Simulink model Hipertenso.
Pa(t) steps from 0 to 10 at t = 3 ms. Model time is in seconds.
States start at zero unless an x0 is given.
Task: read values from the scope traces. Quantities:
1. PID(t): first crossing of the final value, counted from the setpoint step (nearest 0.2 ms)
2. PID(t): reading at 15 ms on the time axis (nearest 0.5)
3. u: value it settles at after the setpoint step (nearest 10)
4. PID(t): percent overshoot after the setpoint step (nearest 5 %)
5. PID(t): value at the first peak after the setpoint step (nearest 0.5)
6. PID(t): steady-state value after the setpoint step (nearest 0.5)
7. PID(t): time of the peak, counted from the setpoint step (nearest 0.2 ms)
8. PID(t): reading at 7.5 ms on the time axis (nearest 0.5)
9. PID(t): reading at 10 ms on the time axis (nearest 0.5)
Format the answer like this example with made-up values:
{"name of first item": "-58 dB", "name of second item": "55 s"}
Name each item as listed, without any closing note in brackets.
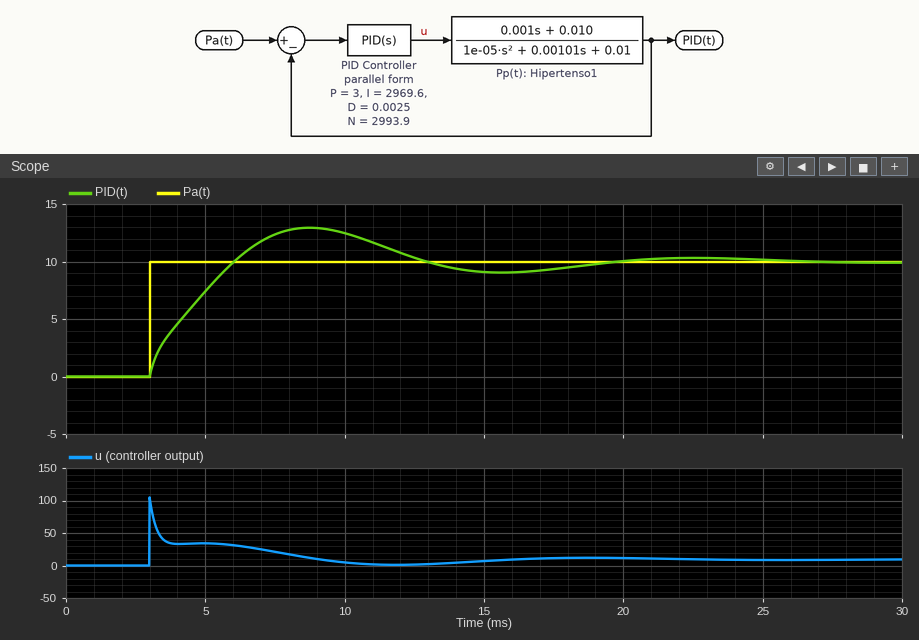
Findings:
{"PID(t): first crossing of the final value, counted from the setpoint step": "3.0 ms", "PID(t): reading at 15 ms on the time axis": "9.0", "u: value it settles at after the setpoint step": "10", "PID(t): percent overshoot after the setpoint step": "30 %", "PID(t): value at the first peak after the setpoint step": "13.0", "PID(t): steady-state value after the setpoint step": "10.0", "PID(t): time of the peak, counted from the setpoint step": "5.8 ms", "PID(t): reading at 7.5 ms on the time axis": "12.5", "PID(t): reading at 10 ms on the time axis": "12.5"}
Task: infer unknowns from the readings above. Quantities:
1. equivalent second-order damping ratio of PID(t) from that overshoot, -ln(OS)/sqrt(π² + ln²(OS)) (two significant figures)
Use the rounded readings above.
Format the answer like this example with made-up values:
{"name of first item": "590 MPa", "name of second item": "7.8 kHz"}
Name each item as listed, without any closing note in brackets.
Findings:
{"equivalent second-order damping ratio of PID(t) from that overshoot, -ln(OS)/sqrt(π² + ln²(OS))": "0.36"}
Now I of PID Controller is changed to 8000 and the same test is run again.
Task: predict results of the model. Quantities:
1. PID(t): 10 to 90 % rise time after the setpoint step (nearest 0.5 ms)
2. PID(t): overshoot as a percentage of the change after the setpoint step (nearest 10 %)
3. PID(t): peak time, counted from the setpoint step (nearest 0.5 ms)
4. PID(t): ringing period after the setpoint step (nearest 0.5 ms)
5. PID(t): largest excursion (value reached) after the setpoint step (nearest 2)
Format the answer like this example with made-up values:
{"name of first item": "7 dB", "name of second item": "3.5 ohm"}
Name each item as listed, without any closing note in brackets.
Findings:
{"PID(t): 10 to 90 % rise time after the setpoint step": "1.5 ms", "PID(t): overshoot as a percentage of the change after the setpoint step": "40 %", "PID(t): peak time, counted from the setpoint step": "3.5 ms", "PID(t): ringing period after the setpoint step": "8.0 ms", "PID(t): largest excursion (value reached) after the setpoint step": "14"}
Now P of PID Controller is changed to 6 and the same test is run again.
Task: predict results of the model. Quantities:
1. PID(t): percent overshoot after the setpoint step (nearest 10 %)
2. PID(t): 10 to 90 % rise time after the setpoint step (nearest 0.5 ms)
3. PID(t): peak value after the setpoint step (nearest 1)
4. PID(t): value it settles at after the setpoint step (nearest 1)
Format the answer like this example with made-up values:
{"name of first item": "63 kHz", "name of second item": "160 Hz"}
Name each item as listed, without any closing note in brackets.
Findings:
{"PID(t): percent overshoot after the setpoint step": "20 %", "PID(t): 10 to 90 % rise time after the setpoint step": "2.0 ms", "PID(t): peak value after the setpoint step": "12", "PID(t): value it settles at after the setpoint step": "10"}
